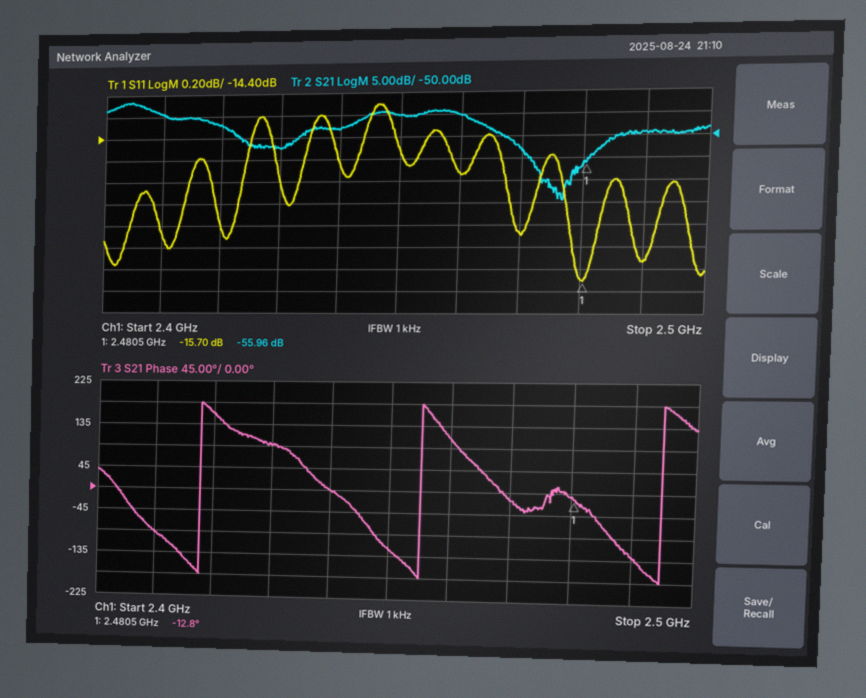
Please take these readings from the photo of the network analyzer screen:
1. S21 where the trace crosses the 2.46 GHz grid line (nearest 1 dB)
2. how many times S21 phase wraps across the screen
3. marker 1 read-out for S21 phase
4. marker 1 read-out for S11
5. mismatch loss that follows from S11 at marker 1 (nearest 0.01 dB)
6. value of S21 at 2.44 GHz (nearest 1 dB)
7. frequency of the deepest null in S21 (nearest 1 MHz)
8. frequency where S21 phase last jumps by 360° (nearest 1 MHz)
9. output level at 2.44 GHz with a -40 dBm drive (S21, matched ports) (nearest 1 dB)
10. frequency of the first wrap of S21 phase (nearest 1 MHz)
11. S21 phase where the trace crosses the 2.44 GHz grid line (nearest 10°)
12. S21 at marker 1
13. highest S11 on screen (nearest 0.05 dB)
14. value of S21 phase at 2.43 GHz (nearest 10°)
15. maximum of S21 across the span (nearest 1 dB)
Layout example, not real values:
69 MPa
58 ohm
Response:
-45 dB
3
-12.8°
-15.70 dB
0.12 dB
-48 dB
2.477 GHz
2.495 GHz
-88 dBm
2.418 GHz
0°
-55.96 dB
-14.10 dB
90°
-42 dB
